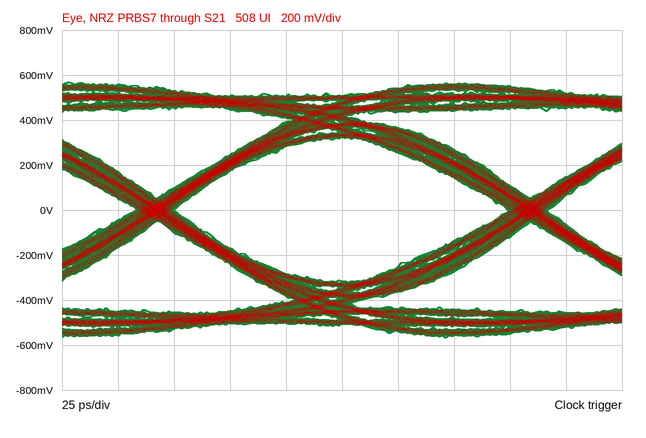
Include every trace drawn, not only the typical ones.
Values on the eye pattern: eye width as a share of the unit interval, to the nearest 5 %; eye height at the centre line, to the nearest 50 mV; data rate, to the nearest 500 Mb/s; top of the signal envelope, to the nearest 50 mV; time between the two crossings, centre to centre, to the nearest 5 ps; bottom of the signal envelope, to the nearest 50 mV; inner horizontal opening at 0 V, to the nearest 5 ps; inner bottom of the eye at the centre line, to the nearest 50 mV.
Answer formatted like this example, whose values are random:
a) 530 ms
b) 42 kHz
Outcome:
a) 90 %
b) 650 mV
c) 6.0 Gb/s
d) 550 mV
e) 165 ps
f) -550 mV
g) 150 ps
h) -300 mV
